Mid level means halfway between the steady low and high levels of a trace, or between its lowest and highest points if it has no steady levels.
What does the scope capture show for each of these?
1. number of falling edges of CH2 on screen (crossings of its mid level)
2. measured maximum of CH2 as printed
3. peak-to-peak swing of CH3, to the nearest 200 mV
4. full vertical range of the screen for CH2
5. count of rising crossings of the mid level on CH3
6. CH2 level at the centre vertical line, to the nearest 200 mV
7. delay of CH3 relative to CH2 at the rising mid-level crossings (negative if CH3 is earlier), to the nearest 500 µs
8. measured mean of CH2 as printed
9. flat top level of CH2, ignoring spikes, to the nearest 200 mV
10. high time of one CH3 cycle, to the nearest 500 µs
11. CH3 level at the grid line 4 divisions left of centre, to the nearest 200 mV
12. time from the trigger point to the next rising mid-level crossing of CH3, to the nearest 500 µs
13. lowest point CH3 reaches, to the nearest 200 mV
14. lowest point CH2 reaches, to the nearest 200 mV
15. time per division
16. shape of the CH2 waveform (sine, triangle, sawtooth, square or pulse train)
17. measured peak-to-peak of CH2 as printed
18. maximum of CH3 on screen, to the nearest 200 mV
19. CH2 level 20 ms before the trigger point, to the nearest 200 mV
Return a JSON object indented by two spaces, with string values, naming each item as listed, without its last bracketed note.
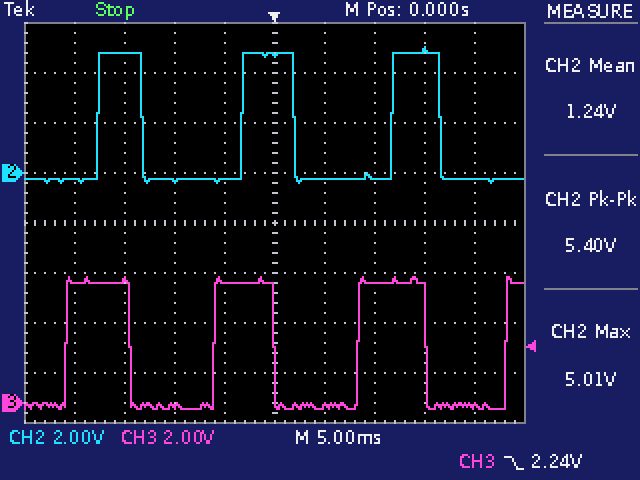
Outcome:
{
  "number of falling edges of CH2 on screen": "3",
  "measured maximum of CH2 as printed": "5.01 V",
  "peak-to-peak swing of CH3, to the nearest 200 mV": "5.2 V",
  "full vertical range of the screen for CH2": "16 V",
  "count of rising crossings of the mid level on CH3": "4",
  "CH2 level at the centre vertical line, to the nearest 200 mV": "4.8 V",
  "delay of CH3 relative to CH2 at the rising mid-level crossings (negative if CH3 is earlier), to the nearest 500 µs": "-3.0 ms",
  "measured mean of CH2 as printed": "1.24 V",
  "flat top level of CH2, ignoring spikes, to the nearest 200 mV": "4.8 V",
  "high time of one CH3 cycle, to the nearest 500 µs": "6.5 ms",
  "CH3 level at the grid line 4 divisions left of centre, to the nearest 200 mV": "4.8 V",
  "time from the trigger point to the next rising mid-level crossing of CH3, to the nearest 500 µs": "8.5 ms",
  "lowest point CH3 reaches, to the nearest 200 mV": "-200 mV",
  "lowest point CH2 reaches, to the nearest 200 mV": "-400 mV",
  "time per division": "5 ms",
  "shape of the CH2 waveform": "pulse train",
  "measured peak-to-peak of CH2 as printed": "5.40 V",
  "maximum of CH3 on screen, to the nearest 200 mV": "5.0 V",
  "CH2 level 20 ms before the trigger point, to the nearest 200 mV": "-200 mV"
}
